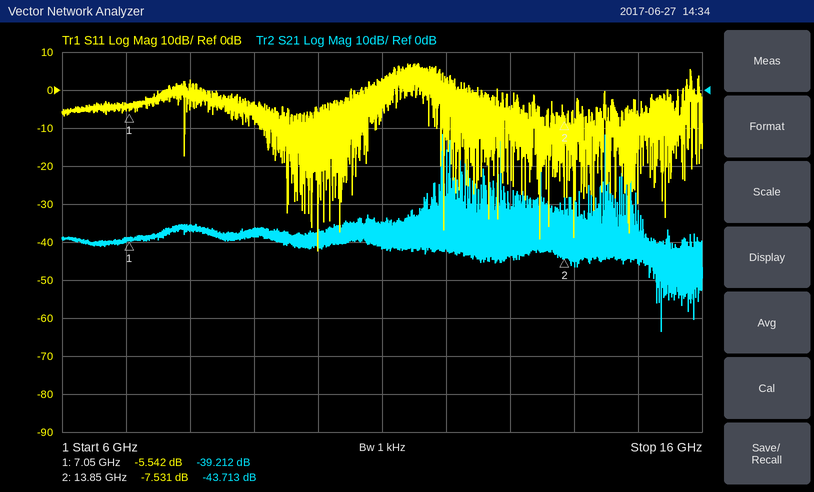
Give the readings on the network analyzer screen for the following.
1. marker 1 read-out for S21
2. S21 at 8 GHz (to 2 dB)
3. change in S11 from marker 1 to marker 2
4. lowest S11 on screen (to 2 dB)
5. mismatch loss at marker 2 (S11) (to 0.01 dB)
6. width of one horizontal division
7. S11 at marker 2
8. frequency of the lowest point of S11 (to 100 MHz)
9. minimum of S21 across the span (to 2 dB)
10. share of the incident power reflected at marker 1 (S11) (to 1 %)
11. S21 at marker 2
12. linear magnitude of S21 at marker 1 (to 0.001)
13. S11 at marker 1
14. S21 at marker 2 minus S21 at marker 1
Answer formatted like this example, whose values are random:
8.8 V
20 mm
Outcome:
-39.212 dB
-36 dB
-1.989 dB
-42 dB
0.84 dB
1 GHz
-7.531 dB
10.0 GHz
-64 dB
28 %
-43.713 dB
0.011
-5.542 dB
-4.501 dB
